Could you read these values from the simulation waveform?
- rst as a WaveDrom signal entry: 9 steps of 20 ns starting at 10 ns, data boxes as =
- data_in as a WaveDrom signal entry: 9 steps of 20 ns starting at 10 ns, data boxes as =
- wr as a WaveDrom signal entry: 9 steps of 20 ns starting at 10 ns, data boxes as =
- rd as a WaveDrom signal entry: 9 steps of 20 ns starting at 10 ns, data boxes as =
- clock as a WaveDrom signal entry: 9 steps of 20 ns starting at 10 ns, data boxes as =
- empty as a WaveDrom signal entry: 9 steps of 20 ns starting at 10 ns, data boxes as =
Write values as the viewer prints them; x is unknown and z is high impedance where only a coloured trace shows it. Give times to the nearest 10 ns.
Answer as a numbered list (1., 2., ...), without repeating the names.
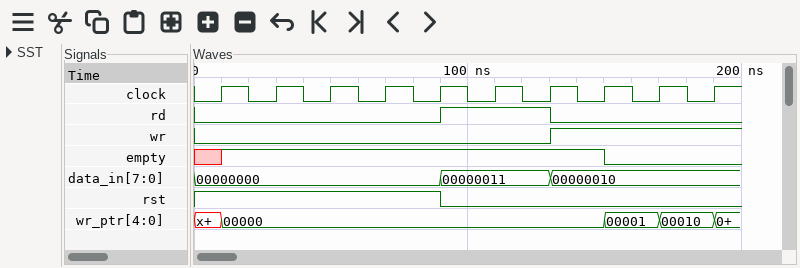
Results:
1. {name: 'rst', wave: '1...0....'}
2. {name: 'data_in', wave: '=...=.=..', data: '00000000 00000011 00000010'}
3. {name: 'wr', wave: '0.....1..'}
4. {name: 'rd', wave: '0...1.0..'}
5. {name: 'clock', wave: 'p........'}
6. {name: 'empty', wave: '1......0.'}
